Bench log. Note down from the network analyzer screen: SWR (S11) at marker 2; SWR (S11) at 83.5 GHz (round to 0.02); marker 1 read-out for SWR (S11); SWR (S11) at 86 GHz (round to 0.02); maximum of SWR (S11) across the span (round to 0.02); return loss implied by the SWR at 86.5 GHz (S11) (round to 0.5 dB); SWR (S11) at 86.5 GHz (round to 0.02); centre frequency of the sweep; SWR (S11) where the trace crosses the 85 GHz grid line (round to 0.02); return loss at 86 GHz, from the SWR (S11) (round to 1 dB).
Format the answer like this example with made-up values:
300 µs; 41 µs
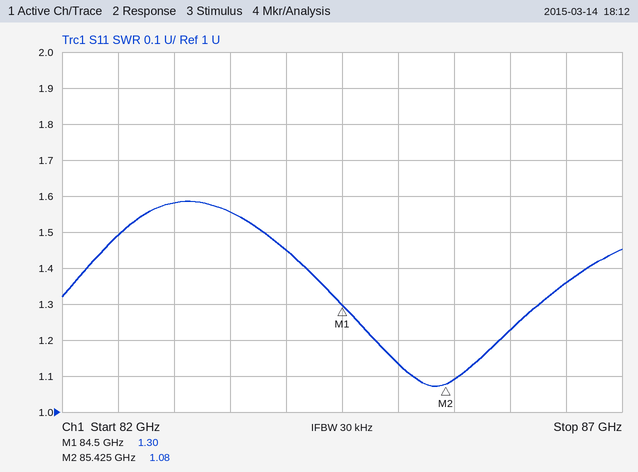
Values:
1.08; 1.56; 1.30; 1.22; 1.58; 16.5 dB; 1.36; 84.5 GHz; 1.14; 20 dB
